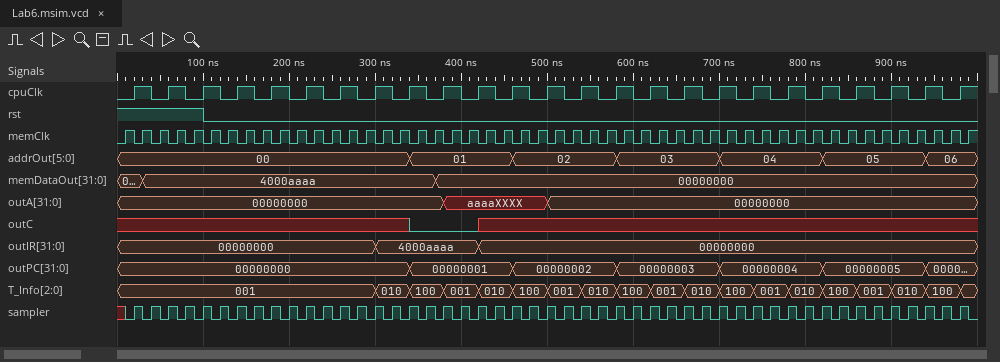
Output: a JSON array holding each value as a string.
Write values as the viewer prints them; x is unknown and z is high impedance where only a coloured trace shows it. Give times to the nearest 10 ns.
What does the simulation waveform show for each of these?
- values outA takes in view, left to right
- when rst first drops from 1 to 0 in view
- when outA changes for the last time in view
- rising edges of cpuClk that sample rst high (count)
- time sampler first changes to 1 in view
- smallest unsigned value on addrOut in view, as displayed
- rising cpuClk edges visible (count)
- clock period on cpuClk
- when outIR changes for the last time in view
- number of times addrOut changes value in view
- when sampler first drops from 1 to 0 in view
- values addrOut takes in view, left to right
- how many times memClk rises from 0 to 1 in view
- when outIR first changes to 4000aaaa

["00000000, aaaaXXXX, 00000000", "100 ns", "500 ns", "3", "20 ns", "00", "25", "40 ns", "420 ns", "6", "30 ns", "00, 01, 02, 03, 04, 05, 06", "50", "300 ns"]
